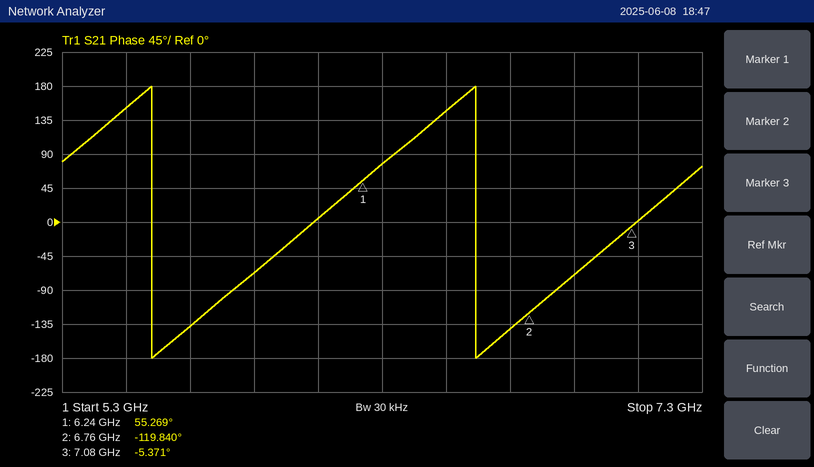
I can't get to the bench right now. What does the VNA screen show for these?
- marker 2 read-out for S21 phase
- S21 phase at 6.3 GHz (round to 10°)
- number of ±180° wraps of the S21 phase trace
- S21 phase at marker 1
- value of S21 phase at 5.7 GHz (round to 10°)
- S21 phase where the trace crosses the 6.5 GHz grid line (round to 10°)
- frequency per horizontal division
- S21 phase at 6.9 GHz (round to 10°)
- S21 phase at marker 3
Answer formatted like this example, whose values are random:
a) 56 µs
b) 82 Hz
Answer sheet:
a) -119.840°
b) 80°
c) 2
d) 55.269°
e) -140°
f) 150°
g) 200 MHz
h) -70°
i) -5.371°
